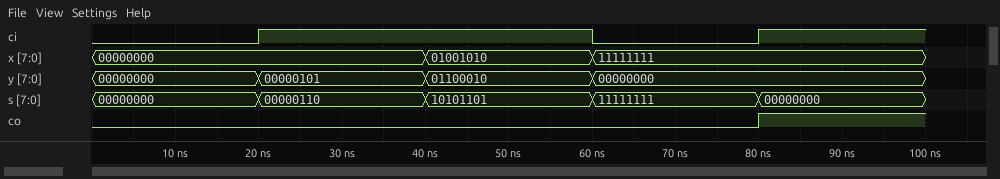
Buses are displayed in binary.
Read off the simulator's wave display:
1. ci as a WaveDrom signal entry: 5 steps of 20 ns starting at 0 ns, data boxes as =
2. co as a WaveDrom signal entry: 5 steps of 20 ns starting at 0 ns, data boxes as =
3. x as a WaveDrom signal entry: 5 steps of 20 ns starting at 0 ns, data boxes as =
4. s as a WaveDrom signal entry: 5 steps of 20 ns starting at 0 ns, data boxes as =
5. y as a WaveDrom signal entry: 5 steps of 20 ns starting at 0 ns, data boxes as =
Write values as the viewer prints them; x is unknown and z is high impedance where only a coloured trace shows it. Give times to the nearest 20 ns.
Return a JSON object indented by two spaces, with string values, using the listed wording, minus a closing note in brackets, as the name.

{
  "ci as a WaveDrom signal entry: 5 steps of 20 ns starting at 0 ns, data boxes as =": "{name: 'ci', wave: '01.01'}",
  "co as a WaveDrom signal entry: 5 steps of 20 ns starting at 0 ns, data boxes as =": "{name: 'co', wave: '0...1'}",
  "x as a WaveDrom signal entry: 5 steps of 20 ns starting at 0 ns, data boxes as =": "{name: 'x', wave: '=.==.', data: '00000000 01001010 11111111'}",
  "s as a WaveDrom signal entry: 5 steps of 20 ns starting at 0 ns, data boxes as =": "{name: 's', wave: '=====', data: '00000000 00000110 10101101 11111111 00000000'}",
  "y as a WaveDrom signal entry: 5 steps of 20 ns starting at 0 ns, data boxes as =": "{name: 'y', wave: '====.', data: '00000000 00000101 01100010 00000000'}"
}
